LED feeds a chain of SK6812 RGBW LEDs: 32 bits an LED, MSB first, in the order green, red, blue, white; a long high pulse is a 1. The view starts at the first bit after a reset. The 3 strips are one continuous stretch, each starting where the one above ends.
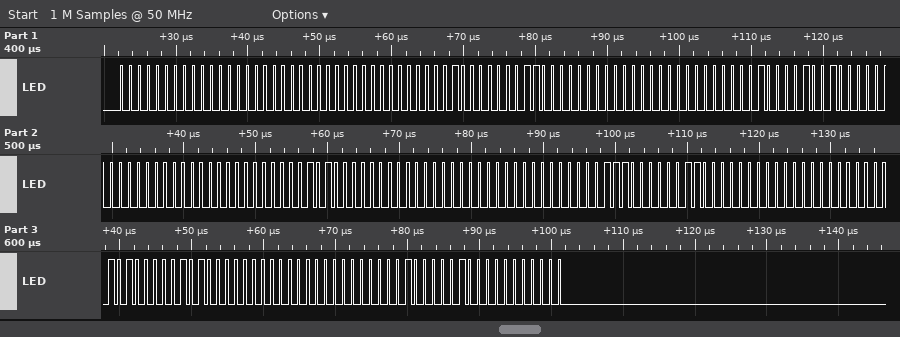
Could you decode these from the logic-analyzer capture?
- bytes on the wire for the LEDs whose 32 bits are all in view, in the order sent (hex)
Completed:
00 00 00 00 04 06 00 00 01 09 00 00 00 0A 00 00 00 07 03 00 00 05 05 00 00 02 08 00
